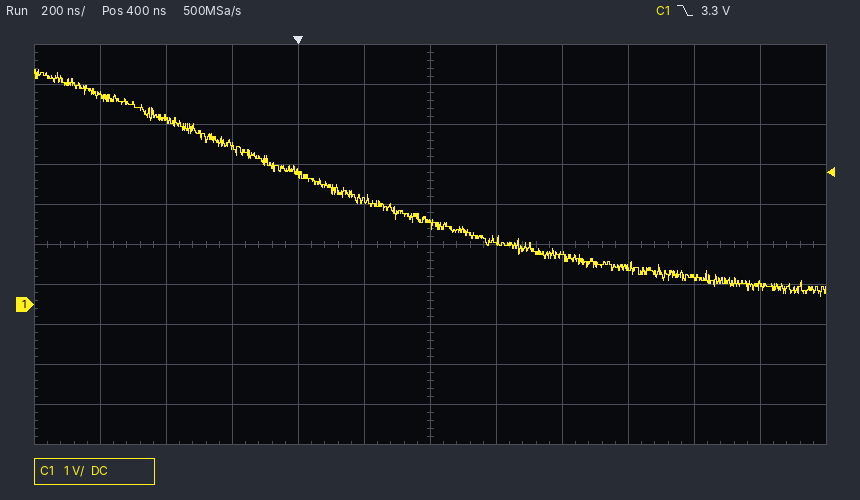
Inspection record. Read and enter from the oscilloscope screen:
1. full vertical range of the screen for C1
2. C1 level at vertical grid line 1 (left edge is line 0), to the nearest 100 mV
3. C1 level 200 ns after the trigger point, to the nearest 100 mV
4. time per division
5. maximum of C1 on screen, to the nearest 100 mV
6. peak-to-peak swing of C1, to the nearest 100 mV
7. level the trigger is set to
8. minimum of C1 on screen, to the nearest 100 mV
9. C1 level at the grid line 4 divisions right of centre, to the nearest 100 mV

10 V
5.2 V
2.6 V
200 ns
5.9 V
5.7 V
3.3 V
200 mV
700 mV
